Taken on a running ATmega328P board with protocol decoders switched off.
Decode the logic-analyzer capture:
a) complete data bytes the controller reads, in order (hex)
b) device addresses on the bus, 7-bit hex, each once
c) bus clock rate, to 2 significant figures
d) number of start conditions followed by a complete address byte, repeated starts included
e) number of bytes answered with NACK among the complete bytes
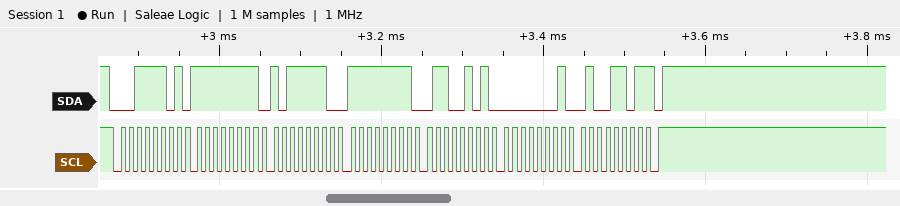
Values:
FF BE FF 65 01 4D
0x1E
100 kHz
1
1
